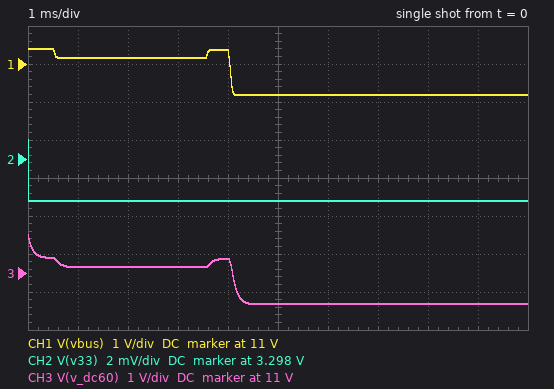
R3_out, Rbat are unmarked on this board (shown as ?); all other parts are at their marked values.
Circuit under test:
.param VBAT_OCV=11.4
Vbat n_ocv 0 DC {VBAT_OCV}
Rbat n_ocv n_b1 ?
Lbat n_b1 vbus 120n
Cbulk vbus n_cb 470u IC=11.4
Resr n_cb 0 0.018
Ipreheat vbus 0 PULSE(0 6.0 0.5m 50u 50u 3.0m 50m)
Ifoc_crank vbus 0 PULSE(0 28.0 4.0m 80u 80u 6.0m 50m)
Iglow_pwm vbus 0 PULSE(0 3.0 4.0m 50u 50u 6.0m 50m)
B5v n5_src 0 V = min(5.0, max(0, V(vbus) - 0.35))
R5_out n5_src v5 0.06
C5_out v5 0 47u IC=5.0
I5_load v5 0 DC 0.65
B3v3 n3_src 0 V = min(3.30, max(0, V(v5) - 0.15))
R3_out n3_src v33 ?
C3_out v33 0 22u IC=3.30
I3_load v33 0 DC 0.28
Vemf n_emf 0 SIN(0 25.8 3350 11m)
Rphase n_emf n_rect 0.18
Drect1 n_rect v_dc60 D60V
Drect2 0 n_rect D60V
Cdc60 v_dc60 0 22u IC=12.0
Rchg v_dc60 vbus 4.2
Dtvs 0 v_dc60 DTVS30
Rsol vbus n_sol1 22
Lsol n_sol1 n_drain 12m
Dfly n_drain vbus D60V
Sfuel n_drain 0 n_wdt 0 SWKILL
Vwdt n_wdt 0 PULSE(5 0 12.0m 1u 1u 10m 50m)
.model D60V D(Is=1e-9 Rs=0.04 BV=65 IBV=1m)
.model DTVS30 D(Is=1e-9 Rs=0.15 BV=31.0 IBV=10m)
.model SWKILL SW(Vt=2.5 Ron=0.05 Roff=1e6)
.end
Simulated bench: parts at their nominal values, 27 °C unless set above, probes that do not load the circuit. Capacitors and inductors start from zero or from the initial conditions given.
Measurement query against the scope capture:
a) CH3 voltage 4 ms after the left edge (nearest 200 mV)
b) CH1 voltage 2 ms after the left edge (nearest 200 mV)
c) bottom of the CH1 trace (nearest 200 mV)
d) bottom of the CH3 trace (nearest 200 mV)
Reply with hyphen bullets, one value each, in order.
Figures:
- 11.4 V
- 11.2 V
- 10.2 V
- 10.2 V
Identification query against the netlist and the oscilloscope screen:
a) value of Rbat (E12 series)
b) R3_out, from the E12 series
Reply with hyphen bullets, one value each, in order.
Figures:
- 0.039 Ω
- 0.015 Ω
